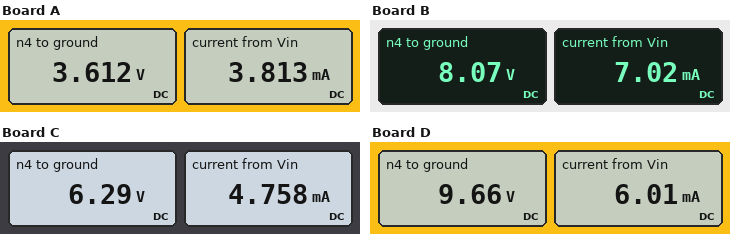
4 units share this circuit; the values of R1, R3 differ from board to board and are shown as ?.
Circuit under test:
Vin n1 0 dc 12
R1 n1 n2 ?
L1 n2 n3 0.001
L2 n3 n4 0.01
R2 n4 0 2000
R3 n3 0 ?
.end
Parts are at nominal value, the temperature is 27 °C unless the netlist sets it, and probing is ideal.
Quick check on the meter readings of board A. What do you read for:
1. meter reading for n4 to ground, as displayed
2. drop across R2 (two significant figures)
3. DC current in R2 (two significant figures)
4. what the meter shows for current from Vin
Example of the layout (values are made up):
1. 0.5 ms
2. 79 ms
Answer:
1. 3.612 V
2. 3.6 V
3. 1.8 mA
4. 3.813 mA
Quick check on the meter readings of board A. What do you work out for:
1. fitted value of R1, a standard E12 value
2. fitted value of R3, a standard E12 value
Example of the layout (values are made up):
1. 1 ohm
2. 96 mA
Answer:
1. 2.2 kΩ
2. 1.8 kΩ
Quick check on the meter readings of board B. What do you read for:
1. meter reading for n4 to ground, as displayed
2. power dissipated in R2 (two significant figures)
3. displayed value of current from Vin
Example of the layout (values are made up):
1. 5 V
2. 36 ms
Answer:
1. 8.07 V
2. 33 mW
3. 7.02 mA
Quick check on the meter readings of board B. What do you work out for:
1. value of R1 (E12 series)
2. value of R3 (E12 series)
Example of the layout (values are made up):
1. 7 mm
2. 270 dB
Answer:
1. 560 Ω
2. 2.7 kΩ
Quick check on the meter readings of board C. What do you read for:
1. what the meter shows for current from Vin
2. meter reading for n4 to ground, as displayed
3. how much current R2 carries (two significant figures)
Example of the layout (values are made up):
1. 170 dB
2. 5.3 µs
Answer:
1. 4.758 mA
2. 6.29 V
3. 3.1 mA
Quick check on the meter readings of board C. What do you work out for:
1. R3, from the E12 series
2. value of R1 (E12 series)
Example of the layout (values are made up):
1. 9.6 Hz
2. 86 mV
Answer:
1. 3.9 kΩ
2. 1.2 kΩ
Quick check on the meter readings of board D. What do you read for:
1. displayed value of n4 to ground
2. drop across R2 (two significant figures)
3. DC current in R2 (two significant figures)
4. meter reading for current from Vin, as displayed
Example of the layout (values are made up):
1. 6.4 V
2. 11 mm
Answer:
1. 9.66 V
2. 9.7 V
3. 4.8 mA
4. 6.01 mA
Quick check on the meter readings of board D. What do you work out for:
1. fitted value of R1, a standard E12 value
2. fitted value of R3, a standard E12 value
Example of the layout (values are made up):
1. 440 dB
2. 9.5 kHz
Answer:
1. 390 Ω
2. 8.2 kΩ
